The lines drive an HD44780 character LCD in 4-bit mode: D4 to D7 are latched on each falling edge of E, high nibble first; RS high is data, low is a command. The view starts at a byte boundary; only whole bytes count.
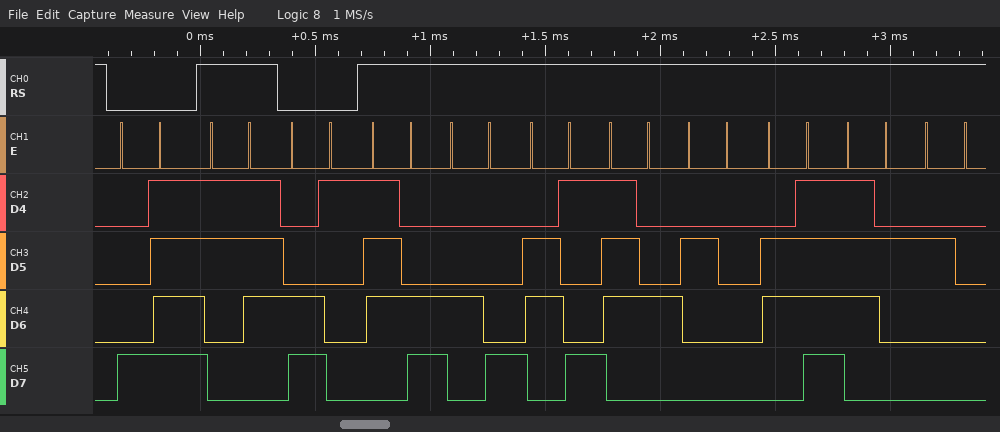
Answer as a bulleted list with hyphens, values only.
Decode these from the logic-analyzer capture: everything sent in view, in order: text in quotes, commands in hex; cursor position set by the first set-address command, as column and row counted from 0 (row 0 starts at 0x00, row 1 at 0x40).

- 0x8F "7" 0xC1 "|Hit or "
- column 15, row 0
